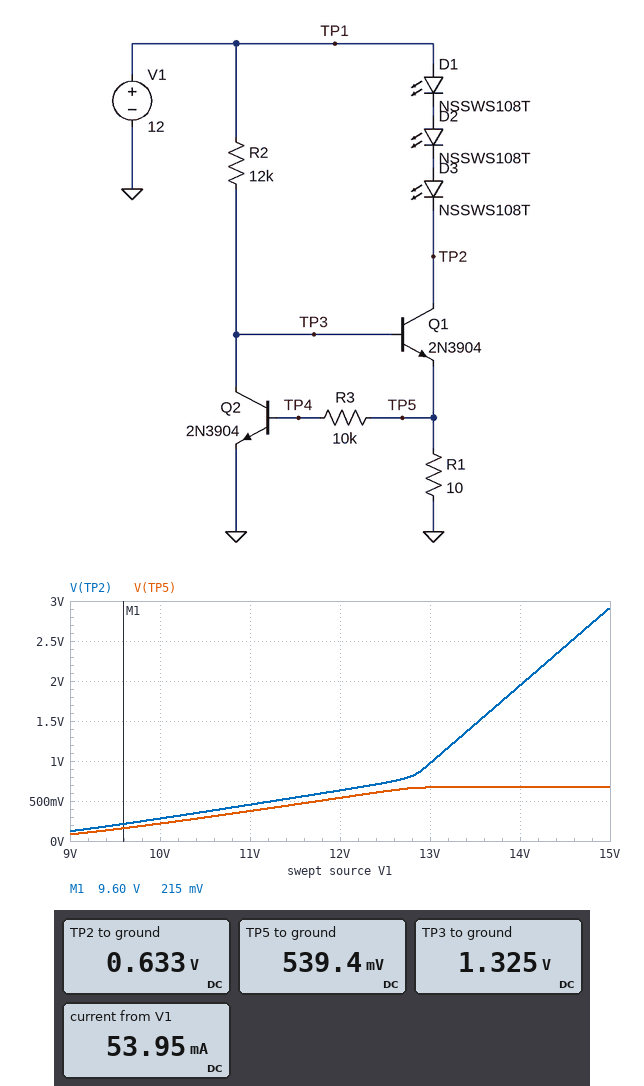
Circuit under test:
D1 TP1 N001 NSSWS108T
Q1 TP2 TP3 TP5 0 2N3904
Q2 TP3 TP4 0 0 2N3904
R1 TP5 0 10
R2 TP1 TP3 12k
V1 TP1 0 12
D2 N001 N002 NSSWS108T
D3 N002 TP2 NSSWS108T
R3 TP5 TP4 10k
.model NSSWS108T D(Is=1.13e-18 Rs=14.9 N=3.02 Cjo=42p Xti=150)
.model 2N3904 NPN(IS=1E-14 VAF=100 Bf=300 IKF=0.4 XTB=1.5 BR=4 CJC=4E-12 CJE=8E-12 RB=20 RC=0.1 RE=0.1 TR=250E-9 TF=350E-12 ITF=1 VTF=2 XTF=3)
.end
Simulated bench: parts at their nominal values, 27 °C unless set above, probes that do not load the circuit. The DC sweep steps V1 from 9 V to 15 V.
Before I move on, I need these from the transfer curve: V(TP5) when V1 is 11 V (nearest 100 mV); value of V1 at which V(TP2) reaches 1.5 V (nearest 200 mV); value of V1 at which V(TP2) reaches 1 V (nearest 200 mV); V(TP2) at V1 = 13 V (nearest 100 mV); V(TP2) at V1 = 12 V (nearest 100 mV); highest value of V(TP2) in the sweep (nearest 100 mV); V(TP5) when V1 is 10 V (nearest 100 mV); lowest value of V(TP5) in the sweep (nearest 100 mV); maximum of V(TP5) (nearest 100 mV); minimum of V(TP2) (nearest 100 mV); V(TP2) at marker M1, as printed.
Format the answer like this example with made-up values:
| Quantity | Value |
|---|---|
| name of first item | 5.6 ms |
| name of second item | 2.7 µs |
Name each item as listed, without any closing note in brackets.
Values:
| Quantity | Value |
|---|---|
| V(TP5) when V1 is 11 V | 400 mV |
| value of V1 at which V(TP2) reaches 1.5 V | 13.6 V |
| value of V1 at which V(TP2) reaches 1 V | 13.0 V |
| V(TP2) at V1 = 13 V | 1.0 V |
| V(TP2) at V1 = 12 V | 600 mV |
| highest value of V(TP2) in the sweep | 2.9 V |
| V(TP5) when V1 is 10 V | 200 mV |
| lowest value of V(TP5) in the sweep | 100 mV |
| maximum of V(TP5) | 700 mV |
| minimum of V(TP2) | 100 mV |
| V(TP2) at marker M1, as printed | 215 mV |
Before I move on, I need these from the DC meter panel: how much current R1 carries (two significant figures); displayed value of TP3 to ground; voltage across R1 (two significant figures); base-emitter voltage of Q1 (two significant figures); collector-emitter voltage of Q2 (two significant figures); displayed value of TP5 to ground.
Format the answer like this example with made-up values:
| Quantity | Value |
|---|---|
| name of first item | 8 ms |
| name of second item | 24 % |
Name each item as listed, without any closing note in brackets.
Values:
| Quantity | Value |
|---|---|
| how much current R1 carries | 54 mA |
| displayed value of TP3 to ground | 1.325 V |
| voltage across R1 | 540 mV |
| base-emitter voltage of Q1 | 790 mV |
| collector-emitter voltage of Q2 | 1.3 V |
| displayed value of TP5 to ground | 539.4 mV |
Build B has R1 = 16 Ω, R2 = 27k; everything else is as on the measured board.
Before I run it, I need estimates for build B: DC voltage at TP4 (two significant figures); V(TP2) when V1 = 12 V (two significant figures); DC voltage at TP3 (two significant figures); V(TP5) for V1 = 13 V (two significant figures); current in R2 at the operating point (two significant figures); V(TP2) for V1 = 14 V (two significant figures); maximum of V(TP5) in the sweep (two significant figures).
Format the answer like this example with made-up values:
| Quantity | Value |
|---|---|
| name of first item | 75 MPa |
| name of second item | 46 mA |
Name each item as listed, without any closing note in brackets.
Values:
| Quantity | Value |
|---|---|
| DC voltage at TP4 | 620 mV |
| V(TP2) when V1 = 12 V | 1.3 V |
| DC voltage at TP3 | 1.4 V |
| V(TP5) for V1 = 13 V | 630 mV |
| current in R2 at the operating point | 390 µA |
| V(TP2) for V1 = 14 V | 3.3 V |
| maximum of V(TP5) in the sweep | 640 mV |
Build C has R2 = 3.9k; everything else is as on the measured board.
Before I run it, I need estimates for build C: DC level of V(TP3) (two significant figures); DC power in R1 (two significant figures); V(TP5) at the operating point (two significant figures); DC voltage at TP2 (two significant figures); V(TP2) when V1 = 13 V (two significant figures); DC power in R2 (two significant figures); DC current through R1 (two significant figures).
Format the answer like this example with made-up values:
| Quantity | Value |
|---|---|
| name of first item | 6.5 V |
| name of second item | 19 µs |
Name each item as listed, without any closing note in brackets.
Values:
| Quantity | Value |
|---|---|
| DC level of V(TP3) | 1.4 V |
| DC power in R1 | 31 mW |
| V(TP5) at the operating point | 560 mV |
| DC voltage at TP2 | 620 mV |
| V(TP2) when V1 = 13 V | 810 mV |
| DC power in R2 | 29 mW |
| DC current through R1 | 56 mA |
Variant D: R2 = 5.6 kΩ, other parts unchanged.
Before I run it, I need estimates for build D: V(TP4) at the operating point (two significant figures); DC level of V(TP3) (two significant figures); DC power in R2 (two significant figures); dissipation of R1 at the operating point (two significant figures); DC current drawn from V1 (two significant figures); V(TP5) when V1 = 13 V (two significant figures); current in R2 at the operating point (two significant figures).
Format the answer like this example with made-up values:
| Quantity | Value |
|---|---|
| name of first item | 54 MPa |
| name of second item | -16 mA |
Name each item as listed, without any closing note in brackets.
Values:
| Quantity | Value |
|---|---|
| V(TP4) at the operating point | 550 mV |
| DC level of V(TP3) | 1.4 V |
| DC power in R2 | 20 mW |
| dissipation of R1 at the operating point | 30 mW |
| DC current drawn from V1 | 55 mA |
| V(TP5) when V1 = 13 V | 710 mV |
| current in R2 at the operating point | 1.9 mA |
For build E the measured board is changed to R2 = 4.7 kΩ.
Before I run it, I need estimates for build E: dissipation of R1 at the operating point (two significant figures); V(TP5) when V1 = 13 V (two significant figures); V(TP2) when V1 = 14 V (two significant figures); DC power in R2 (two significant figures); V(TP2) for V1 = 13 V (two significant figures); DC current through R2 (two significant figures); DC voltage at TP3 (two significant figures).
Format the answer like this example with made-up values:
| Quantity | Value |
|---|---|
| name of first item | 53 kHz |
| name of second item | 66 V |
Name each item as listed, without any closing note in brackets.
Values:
| Quantity | Value |
|---|---|
| dissipation of R1 at the operating point | 31 mW |
| V(TP5) when V1 = 13 V | 710 mV |
| V(TP2) when V1 = 14 V | 1.6 V |
| DC power in R2 | 24 mW |
| V(TP2) for V1 = 13 V | 810 mV |
| DC current through R2 | 2.3 mA |
| DC voltage at TP3 | 1.4 V |
